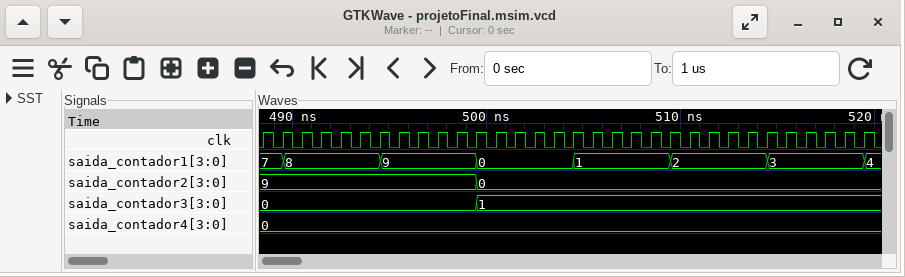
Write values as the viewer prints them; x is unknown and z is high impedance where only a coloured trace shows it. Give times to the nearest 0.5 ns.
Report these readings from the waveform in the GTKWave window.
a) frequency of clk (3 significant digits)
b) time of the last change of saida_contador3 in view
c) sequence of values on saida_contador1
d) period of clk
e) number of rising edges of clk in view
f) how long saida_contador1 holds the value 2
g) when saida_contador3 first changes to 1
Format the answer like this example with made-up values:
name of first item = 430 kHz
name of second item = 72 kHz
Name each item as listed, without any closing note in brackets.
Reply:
frequency of clk = 1.00 GHz
time of the last change of saida_contador3 in view = 499.5 ns
sequence of values on saida_contador1 = 7, 8, 9, 0, 1, 2, 3, 4
period of clk = 1 ns
number of rising edges of clk in view = 32
how long saida_contador1 holds the value 2 = 5 ns
when saida_contador3 first changes to 1 = 499.5 ns
